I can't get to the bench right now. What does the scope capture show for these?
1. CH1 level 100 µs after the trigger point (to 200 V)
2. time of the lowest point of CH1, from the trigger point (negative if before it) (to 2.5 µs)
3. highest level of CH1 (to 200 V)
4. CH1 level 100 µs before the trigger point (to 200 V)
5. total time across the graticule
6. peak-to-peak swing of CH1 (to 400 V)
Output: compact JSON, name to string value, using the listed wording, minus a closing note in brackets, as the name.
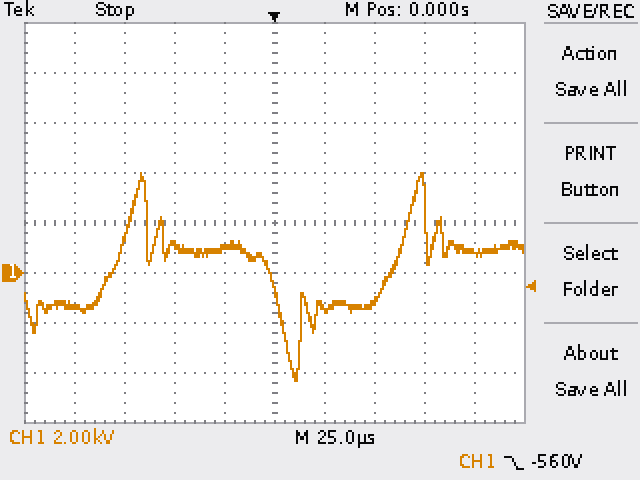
{"CH1 level 100 µs after the trigger point": "800 V", "time of the lowest point of CH1, from the trigger point (negative if before it)": "+10.0 µs", "highest level of CH1": "4.0 kV", "CH1 level 100 µs before the trigger point": "-1.4 kV", "total time across the graticule": "250 µs", "peak-to-peak swing of CH1": "8.4 kV"}
